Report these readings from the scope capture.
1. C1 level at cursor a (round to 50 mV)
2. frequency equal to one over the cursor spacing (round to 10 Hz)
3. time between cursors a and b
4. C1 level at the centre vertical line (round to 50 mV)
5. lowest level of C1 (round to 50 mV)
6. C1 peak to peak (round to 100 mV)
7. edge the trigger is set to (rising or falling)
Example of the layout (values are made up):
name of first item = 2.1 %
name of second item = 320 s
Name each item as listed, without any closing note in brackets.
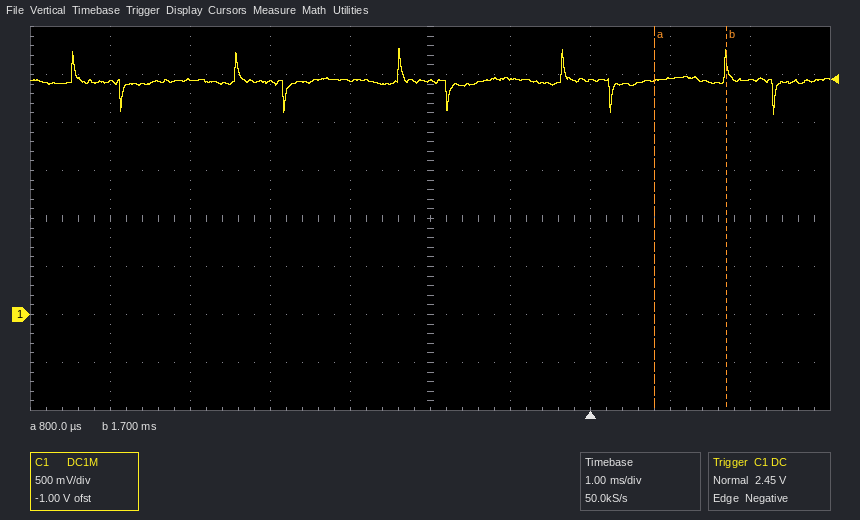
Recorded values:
C1 level at cursor a = 2.45 V
frequency equal to one over the cursor spacing = 1.11 kHz
time between cursors a and b = 900 µs
C1 level at the centre vertical line = 2.45 V
lowest level of C1 = 2.10 V
C1 peak to peak = 700 mV
edge the trigger is set to = falling
